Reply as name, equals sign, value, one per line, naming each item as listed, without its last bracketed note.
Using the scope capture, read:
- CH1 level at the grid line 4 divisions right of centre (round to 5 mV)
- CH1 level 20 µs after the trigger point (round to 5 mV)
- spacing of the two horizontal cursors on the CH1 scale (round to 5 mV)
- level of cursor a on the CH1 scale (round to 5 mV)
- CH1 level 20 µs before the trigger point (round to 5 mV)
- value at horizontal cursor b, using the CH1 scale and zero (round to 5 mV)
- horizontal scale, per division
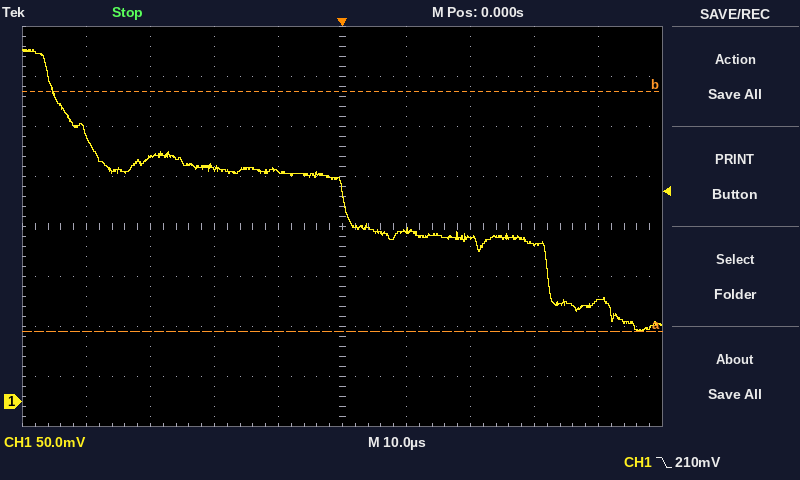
CH1 level at the grid line 4 divisions right of centre = 100 mV
CH1 level 20 µs after the trigger point = 165 mV
spacing of the two horizontal cursors on the CH1 scale = 240 mV
level of cursor a on the CH1 scale = 70 mV
CH1 level 20 µs before the trigger point = 235 mV
value at horizontal cursor b, using the CH1 scale and zero = 310 mV
horizontal scale, per division = 10 µs
